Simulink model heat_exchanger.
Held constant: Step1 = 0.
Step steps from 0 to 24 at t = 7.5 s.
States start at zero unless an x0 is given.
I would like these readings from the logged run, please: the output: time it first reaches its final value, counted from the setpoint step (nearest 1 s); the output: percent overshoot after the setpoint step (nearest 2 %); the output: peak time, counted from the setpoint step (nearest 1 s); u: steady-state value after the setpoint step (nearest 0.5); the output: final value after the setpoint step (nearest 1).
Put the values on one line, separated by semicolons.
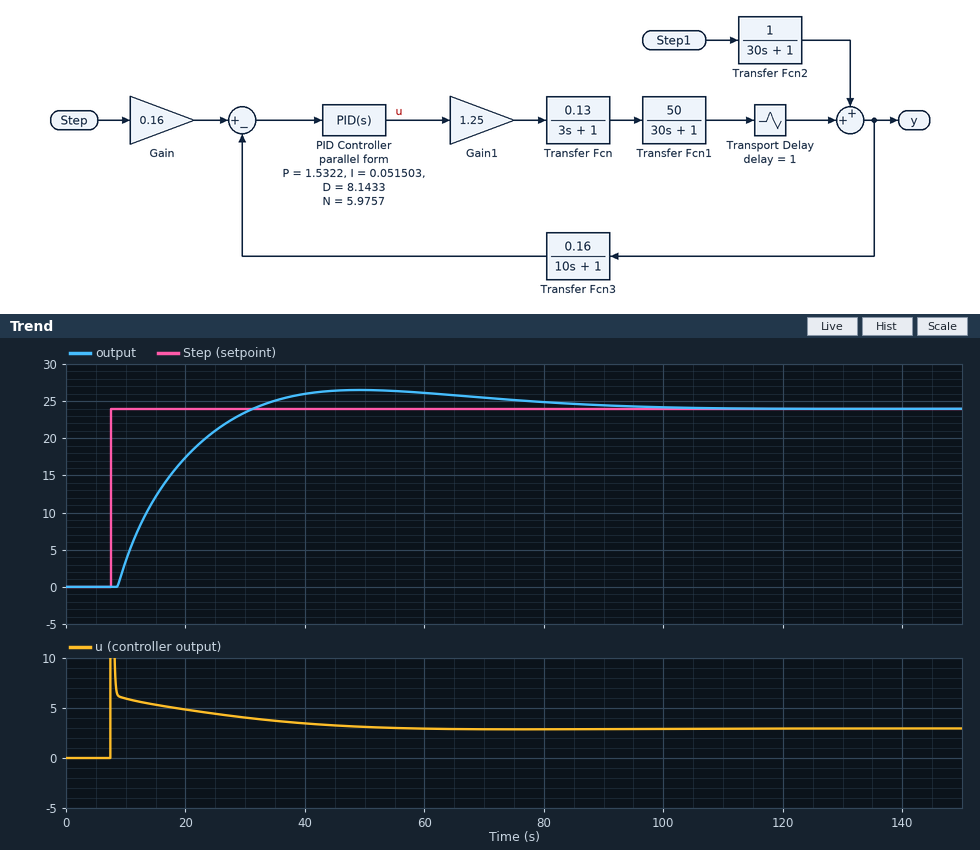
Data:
24 s; 10 %; 42 s; 3.0; 24
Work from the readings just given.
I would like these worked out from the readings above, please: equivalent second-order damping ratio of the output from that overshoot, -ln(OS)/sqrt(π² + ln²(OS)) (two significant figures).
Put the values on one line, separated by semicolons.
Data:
0.59
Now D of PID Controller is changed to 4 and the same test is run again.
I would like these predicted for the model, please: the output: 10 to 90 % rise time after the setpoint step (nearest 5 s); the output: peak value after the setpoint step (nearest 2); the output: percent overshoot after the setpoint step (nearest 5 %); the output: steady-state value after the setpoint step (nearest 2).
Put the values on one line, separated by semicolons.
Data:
15 s; 28; 20 %; 24
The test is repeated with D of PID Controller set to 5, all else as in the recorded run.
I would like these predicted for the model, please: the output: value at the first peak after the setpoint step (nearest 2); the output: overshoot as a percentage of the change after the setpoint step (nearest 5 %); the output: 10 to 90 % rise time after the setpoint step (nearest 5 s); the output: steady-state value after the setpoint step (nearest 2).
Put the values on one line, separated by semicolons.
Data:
28; 15 %; 15 s; 24
